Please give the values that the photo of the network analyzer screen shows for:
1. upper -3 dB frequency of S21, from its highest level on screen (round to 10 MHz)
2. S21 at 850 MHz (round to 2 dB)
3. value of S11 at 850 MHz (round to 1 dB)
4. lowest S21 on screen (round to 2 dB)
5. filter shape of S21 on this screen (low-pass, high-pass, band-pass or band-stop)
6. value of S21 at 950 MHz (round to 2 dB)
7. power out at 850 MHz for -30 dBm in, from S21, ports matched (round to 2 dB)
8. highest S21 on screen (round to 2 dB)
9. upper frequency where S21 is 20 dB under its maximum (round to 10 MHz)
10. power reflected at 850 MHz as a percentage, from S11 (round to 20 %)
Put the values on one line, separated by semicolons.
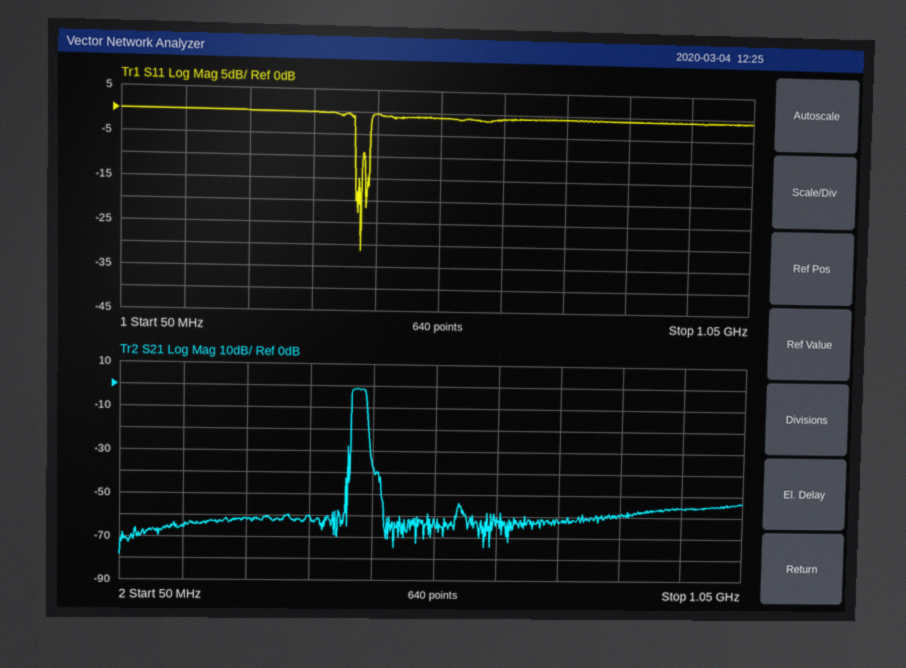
440 MHz; -60 dB; -1 dB; -78 dB; band-pass; -56 dB; -90 dBm; -2 dB; 440 MHz; 80 %
